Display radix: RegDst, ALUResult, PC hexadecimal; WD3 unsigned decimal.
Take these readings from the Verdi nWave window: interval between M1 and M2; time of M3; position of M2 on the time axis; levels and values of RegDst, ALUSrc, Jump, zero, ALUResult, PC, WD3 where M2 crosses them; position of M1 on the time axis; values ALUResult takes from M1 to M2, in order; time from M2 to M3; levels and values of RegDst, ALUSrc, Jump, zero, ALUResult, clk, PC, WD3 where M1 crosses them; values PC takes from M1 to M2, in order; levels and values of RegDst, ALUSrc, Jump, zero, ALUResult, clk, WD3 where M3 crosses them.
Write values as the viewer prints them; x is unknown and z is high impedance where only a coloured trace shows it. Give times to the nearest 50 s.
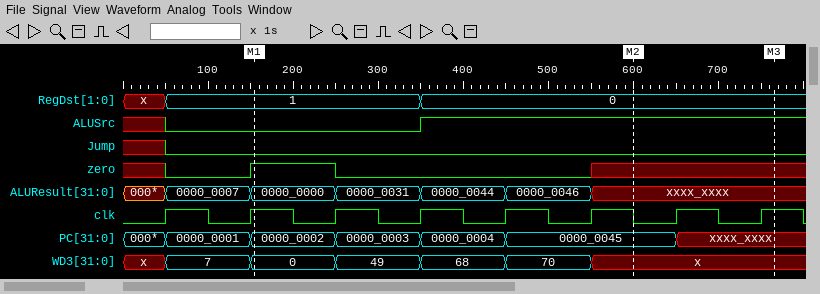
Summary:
450 s
750 s
600 s
RegDst=0, ALUSrc=1, Jump=0, zero=x, ALUResult=xxxx_xxxx, PC=0000_0045, WD3=x
150 s
0000_0000, 0000_0031, 0000_0044, 0000_0046, xxxx_xxxx
150 s
RegDst=1, ALUSrc=0, Jump=0, zero=1, ALUResult=0000_0000, clk=1, PC=0000_0002, WD3=0
0000_0002, 0000_0003, 0000_0004, 0000_0045
RegDst=0, ALUSrc=1, Jump=0, zero=x, ALUResult=xxxx_xxxx, clk=1, WD3=x
